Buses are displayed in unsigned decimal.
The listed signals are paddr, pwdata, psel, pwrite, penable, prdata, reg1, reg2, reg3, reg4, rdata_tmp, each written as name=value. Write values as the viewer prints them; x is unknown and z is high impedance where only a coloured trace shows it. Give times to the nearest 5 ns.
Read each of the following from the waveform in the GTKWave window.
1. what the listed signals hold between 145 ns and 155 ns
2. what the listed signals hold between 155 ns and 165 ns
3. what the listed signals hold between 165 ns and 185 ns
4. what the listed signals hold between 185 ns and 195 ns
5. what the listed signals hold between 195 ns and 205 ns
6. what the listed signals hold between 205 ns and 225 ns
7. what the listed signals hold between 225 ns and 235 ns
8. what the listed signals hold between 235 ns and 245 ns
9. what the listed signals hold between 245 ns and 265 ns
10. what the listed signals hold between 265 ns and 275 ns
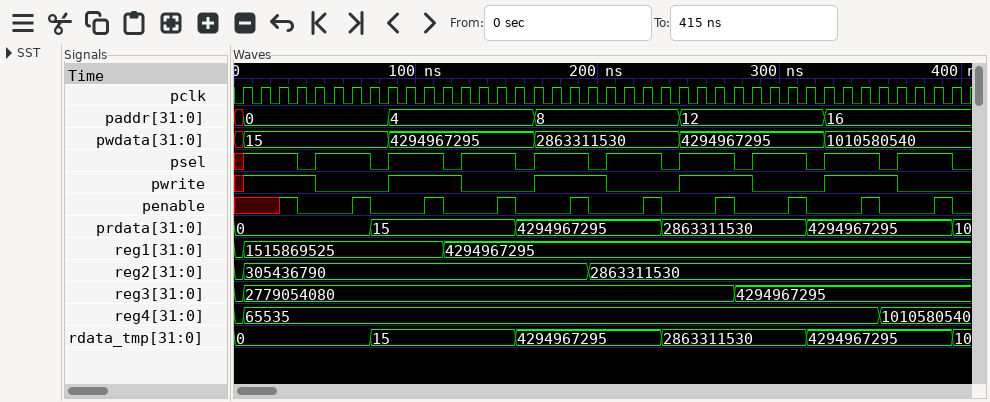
paddr=4, pwdata=4294967295, psel=1, pwrite=0, penable=1, prdata=15, reg1=4294967295, reg2=305436790, reg3=2779054080, reg4=65535, rdata_tmp=15
paddr=4, pwdata=4294967295, psel=0, pwrite=0, penable=0, prdata=4294967295, reg1=4294967295, reg2=305436790, reg3=2779054080, reg4=65535, rdata_tmp=4294967295
paddr=8, pwdata=2863311530, psel=1, pwrite=1, penable=0, prdata=4294967295, reg1=4294967295, reg2=305436790, reg3=2779054080, reg4=65535, rdata_tmp=4294967295
paddr=8, pwdata=2863311530, psel=1, pwrite=1, penable=1, prdata=4294967295, reg1=4294967295, reg2=305436790, reg3=2779054080, reg4=65535, rdata_tmp=4294967295
paddr=8, pwdata=2863311530, psel=0, pwrite=1, penable=0, prdata=4294967295, reg1=4294967295, reg2=2863311530, reg3=2779054080, reg4=65535, rdata_tmp=4294967295
paddr=8, pwdata=2863311530, psel=1, pwrite=0, penable=0, prdata=4294967295, reg1=4294967295, reg2=2863311530, reg3=2779054080, reg4=65535, rdata_tmp=4294967295
paddr=8, pwdata=2863311530, psel=1, pwrite=0, penable=1, prdata=4294967295, reg1=4294967295, reg2=2863311530, reg3=2779054080, reg4=65535, rdata_tmp=4294967295
paddr=8, pwdata=2863311530, psel=0, pwrite=0, penable=0, prdata=2863311530, reg1=4294967295, reg2=2863311530, reg3=2779054080, reg4=65535, rdata_tmp=2863311530
paddr=12, pwdata=4294967295, psel=1, pwrite=1, penable=0, prdata=2863311530, reg1=4294967295, reg2=2863311530, reg3=2779054080, reg4=65535, rdata_tmp=2863311530
paddr=12, pwdata=4294967295, psel=1, pwrite=1, penable=1, prdata=2863311530, reg1=4294967295, reg2=2863311530, reg3=2779054080, reg4=65535, rdata_tmp=2863311530
